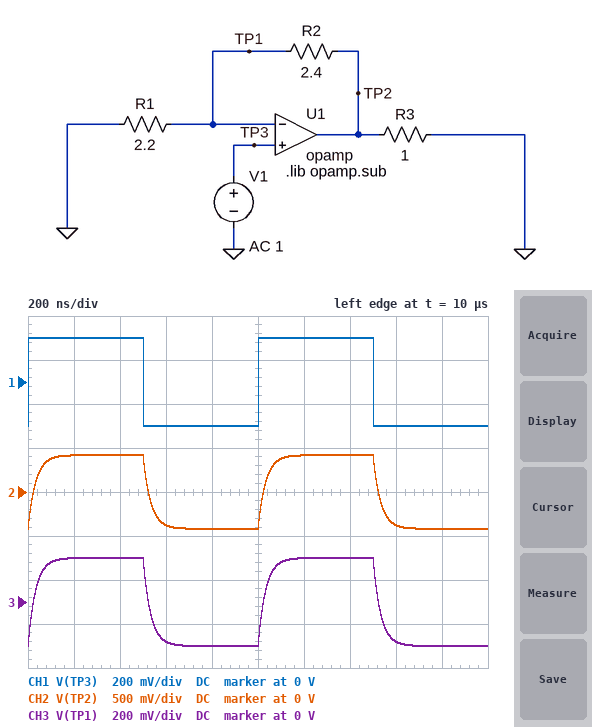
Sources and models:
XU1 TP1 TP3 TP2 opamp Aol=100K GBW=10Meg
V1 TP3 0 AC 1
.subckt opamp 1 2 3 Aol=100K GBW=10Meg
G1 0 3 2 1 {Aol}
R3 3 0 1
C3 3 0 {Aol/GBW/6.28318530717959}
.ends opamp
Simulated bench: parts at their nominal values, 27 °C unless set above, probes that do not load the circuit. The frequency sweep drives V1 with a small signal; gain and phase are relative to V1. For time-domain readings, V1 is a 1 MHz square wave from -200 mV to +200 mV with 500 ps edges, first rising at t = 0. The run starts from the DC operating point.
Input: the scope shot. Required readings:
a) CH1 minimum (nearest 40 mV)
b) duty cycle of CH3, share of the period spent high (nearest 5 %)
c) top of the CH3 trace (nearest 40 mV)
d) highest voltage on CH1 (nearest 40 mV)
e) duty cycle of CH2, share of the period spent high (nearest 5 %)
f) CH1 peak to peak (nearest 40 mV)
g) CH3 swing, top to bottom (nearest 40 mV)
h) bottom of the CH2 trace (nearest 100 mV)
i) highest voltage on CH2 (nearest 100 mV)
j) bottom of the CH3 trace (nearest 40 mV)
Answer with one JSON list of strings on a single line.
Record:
["-200 mV", "50 %", "200 mV", "200 mV", "50 %", "400 mV", "400 mV", "-400 mV", "400 mV", "-200 mV"]
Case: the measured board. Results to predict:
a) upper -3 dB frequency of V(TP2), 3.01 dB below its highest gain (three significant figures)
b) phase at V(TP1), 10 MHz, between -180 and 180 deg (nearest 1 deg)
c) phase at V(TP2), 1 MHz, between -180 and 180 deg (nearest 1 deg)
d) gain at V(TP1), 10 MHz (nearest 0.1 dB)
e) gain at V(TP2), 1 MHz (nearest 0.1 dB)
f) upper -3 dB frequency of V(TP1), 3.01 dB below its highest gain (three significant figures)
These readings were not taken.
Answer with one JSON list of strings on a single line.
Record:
["4.78 MHz", "-64 deg", "-12 deg", "-7.3 dB", "6.2 dB", "4.78 MHz"]
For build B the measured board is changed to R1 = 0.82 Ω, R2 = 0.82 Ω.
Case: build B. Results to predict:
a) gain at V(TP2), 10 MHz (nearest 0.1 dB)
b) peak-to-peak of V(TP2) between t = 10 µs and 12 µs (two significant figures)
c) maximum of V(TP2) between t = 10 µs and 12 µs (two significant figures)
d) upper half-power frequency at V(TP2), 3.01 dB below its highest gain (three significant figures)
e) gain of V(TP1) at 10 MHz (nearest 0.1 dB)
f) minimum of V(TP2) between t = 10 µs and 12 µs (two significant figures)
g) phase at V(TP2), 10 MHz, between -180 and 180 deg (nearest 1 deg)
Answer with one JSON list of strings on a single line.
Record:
["-1.0 dB", "800 mV", "400 mV", "5.00 MHz", "-7.0 dB", "-400 mV", "-63 deg"]
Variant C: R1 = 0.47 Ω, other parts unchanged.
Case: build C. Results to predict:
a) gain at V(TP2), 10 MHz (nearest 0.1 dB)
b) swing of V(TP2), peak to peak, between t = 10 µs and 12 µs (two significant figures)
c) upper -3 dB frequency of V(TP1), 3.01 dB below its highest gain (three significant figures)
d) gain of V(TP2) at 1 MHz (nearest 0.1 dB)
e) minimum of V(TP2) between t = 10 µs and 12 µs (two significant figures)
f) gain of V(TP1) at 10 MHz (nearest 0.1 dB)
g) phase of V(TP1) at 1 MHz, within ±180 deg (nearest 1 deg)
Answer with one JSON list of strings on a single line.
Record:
["-0.1 dB", "2.4 V", "1.64 MHz", "14.3 dB", "-1.2 V", "-15.8 dB", "-31 deg"]
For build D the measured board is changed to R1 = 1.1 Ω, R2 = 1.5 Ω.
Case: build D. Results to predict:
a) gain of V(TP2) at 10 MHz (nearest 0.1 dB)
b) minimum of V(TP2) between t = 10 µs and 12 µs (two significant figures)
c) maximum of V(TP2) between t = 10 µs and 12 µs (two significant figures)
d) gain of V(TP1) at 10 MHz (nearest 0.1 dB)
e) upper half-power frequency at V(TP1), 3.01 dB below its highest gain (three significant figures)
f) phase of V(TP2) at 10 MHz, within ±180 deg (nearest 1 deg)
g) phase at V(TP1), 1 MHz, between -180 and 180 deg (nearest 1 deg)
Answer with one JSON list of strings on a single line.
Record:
["-0.7 dB", "-470 mV", "470 mV", "-8.2 dB", "4.23 MHz", "-67 deg", "-13 deg"]
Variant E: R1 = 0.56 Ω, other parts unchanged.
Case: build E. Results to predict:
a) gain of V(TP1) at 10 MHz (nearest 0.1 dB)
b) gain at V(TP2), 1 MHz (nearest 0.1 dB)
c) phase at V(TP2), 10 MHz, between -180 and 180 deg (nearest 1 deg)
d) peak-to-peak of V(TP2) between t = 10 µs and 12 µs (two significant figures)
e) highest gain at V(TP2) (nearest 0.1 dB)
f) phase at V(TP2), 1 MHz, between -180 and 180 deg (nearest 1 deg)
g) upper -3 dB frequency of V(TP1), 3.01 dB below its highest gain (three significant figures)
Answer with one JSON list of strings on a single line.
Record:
["-14.6 dB", "13.4 dB", "-79 deg", "2.1 V", "14.5 dB", "-28 deg", "1.89 MHz"]
